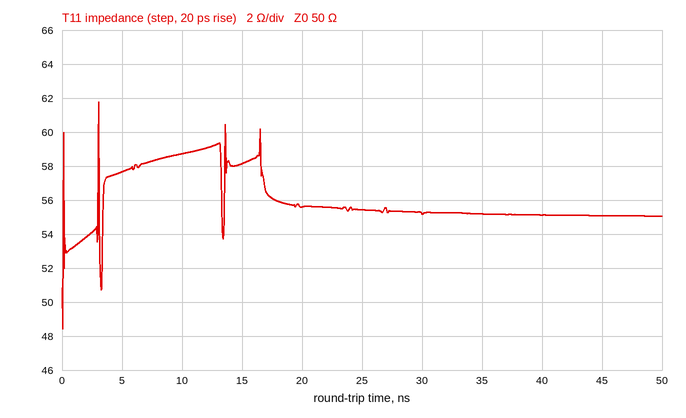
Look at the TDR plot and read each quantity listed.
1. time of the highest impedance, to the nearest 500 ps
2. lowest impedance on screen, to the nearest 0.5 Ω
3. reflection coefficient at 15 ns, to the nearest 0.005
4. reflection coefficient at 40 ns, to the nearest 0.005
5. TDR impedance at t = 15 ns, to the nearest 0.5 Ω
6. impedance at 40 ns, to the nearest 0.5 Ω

3.0 ns
48.5 Ω
+0.075
+0.050
58.0 Ω
55.0 Ω
